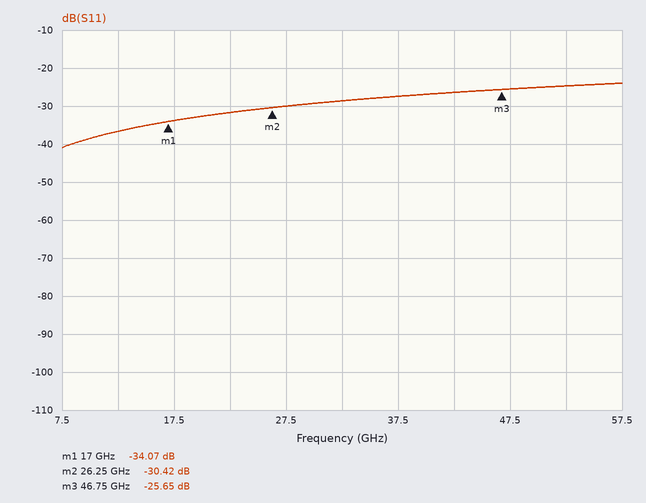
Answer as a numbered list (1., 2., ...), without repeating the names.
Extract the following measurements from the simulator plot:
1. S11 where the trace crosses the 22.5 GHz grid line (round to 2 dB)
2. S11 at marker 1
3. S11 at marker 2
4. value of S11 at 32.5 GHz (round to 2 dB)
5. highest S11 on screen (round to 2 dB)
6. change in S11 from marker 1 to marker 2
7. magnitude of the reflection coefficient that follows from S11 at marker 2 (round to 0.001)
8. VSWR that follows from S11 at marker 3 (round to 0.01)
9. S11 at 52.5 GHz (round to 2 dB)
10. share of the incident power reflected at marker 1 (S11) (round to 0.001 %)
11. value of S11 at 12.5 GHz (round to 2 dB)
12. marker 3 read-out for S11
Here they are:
1. -32 dB
2. -34.07 dB
3. -30.42 dB
4. -28 dB
5. -24 dB
6. 3.65 dB
7. 0.030
8. 1.11
9. -24 dB
10. 0.039 %
11. -36 dB
12. -25.65 dB
